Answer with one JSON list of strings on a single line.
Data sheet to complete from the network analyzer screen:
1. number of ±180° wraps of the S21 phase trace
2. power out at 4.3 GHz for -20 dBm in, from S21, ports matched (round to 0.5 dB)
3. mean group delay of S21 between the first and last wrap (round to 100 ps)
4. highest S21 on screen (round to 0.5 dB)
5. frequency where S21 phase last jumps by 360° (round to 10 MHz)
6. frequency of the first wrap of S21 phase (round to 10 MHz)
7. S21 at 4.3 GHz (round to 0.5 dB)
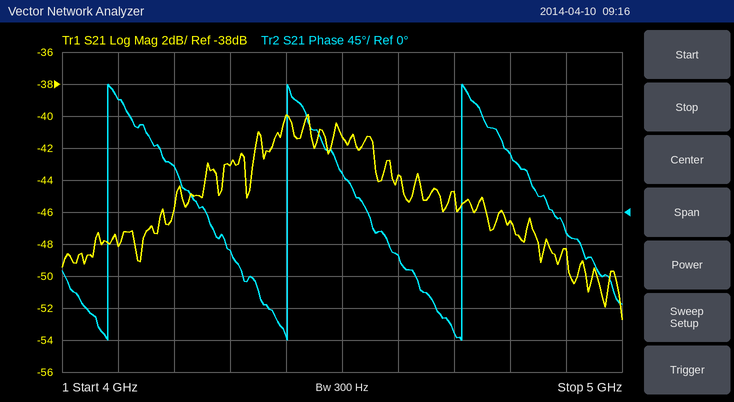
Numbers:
["3", "-63.0 dBm", "3.2 ns", "-40.0 dB", "4.71 GHz", "4.08 GHz", "-43.0 dB"]
